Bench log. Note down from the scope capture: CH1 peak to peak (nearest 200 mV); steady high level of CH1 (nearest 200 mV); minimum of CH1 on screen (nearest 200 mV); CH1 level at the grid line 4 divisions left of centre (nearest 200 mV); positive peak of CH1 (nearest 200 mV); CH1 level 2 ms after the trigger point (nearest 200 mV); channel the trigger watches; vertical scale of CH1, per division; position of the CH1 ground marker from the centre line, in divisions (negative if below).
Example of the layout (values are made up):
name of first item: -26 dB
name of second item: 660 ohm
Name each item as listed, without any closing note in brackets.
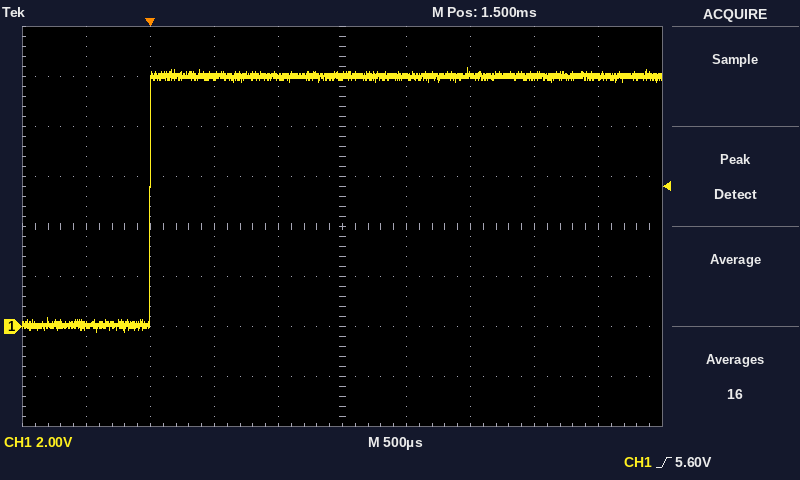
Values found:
CH1 peak to peak: 10.6 V
steady high level of CH1: 10.0 V
minimum of CH1 on screen: -200 mV
CH1 level at the grid line 4 divisions left of centre: 0.0 V
positive peak of CH1: 10.4 V
CH1 level 2 ms after the trigger point: 10.0 V
channel the trigger watches: CH1
vertical scale of CH1, per division: 2 V
position of the CH1 ground marker from the centre line, in divisions: -2.0 div
